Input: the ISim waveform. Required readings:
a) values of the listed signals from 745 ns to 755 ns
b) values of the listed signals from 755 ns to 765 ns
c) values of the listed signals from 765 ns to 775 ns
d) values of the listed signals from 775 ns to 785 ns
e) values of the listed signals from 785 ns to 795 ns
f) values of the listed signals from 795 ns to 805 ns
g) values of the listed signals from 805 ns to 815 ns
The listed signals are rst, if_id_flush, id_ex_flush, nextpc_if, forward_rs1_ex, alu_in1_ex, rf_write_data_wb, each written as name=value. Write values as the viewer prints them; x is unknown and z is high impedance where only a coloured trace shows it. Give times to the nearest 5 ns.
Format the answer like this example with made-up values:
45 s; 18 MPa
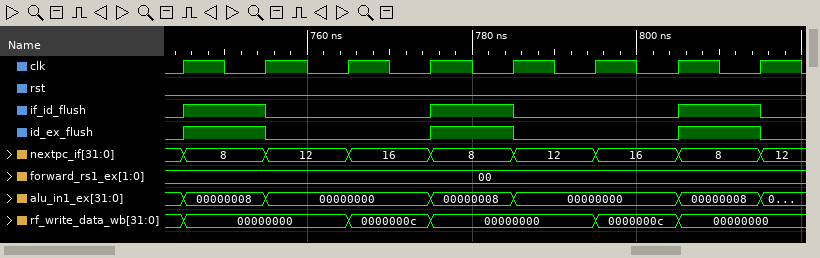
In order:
rst=0, if_id_flush=1, id_ex_flush=1, nextpc_if=8, forward_rs1_ex=00, alu_in1_ex=00000008, rf_write_data_wb=00000000; rst=0, if_id_flush=0, id_ex_flush=0, nextpc_if=12, forward_rs1_ex=00, alu_in1_ex=00000000, rf_write_data_wb=00000000; rst=0, if_id_flush=0, id_ex_flush=0, nextpc_if=16, forward_rs1_ex=00, alu_in1_ex=00000000, rf_write_data_wb=0000000c; rst=0, if_id_flush=1, id_ex_flush=1, nextpc_if=8, forward_rs1_ex=00, alu_in1_ex=00000008, rf_write_data_wb=00000000; rst=0, if_id_flush=0, id_ex_flush=0, nextpc_if=12, forward_rs1_ex=00, alu_in1_ex=00000000, rf_write_data_wb=00000000; rst=0, if_id_flush=0, id_ex_flush=0, nextpc_if=16, forward_rs1_ex=00, alu_in1_ex=00000000, rf_write_data_wb=0000000c; rst=0, if_id_flush=1, id_ex_flush=1, nextpc_if=8, forward_rs1_ex=00, alu_in1_ex=00000008, rf_write_data_wb=00000000
